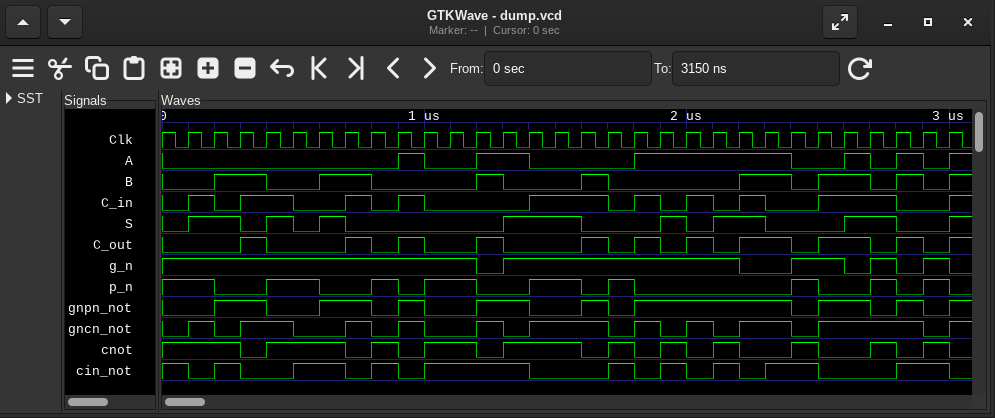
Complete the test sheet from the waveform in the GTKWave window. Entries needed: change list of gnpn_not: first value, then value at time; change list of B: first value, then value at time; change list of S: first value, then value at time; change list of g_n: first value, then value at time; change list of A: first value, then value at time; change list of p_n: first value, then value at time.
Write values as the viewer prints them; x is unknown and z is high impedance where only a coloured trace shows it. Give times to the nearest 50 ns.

0, 1 at 200 ns, 0 at 400 ns, 1 at 600 ns, 0 at 800 ns, 1 at 900 ns, 0 at 1000 ns, 1 at 1200 ns, 0 at 1400 ns, 1 at 1600 ns, 0 at 1700 ns, 1 at 1800 ns, 0 at 2400 ns, 1 at 2500 ns, 0 at 2700 ns, 1 at 2800 ns, 0 at 2900 ns, 1 at 3000 ns
0, 1 at 200 ns, 0 at 400 ns, 1 at 600 ns, 0 at 800 ns, 1 at 1200 ns, 0 at 1300 ns, 1 at 1600 ns, 0 at 1700 ns, 1 at 2200 ns, 0 at 2400 ns, 1 at 2500 ns, 0 at 2700 ns, 1 at 2800 ns, 0 at 2900 ns, 1 at 3000 ns
0, 1 at 100 ns, 0 at 300 ns, 1 at 400 ns, 0 at 500 ns, 1 at 600 ns, 0 at 700 ns, 1 at 1300 ns, 0 at 1600 ns, 1 at 1900 ns, 0 at 2000 ns, 1 at 2100 ns, 0 at 2300 ns, 1 at 2600 ns, 0 at 2800 ns, 1 at 3000 ns
1, 0 at 1200 ns, 1 at 1300 ns, 0 at 2200 ns, 1 at 2400 ns, 0 at 2600 ns, 1 at 2700 ns, 0 at 2800 ns, 1 at 2900 ns, 0 at 3000 ns
0, 1 at 900 ns, 0 at 1000 ns, 1 at 1200 ns, 0 at 1400 ns, 1 at 1800 ns, 0 at 2400 ns, 1 at 2600 ns, 0 at 2700 ns, 1 at 2800 ns, 0 at 2900 ns, 1 at 3000 ns
1, 0 at 200 ns, 1 at 400 ns, 0 at 600 ns, 1 at 800 ns, 0 at 900 ns, 1 at 1000 ns, 0 at 1200 ns, 1 at 1400 ns, 0 at 1600 ns, 1 at 1700 ns, 0 at 1800 ns, 1 at 2400 ns, 0 at 2500 ns, 1 at 2700 ns, 0 at 2800 ns, 1 at 2900 ns, 0 at 3000 ns
